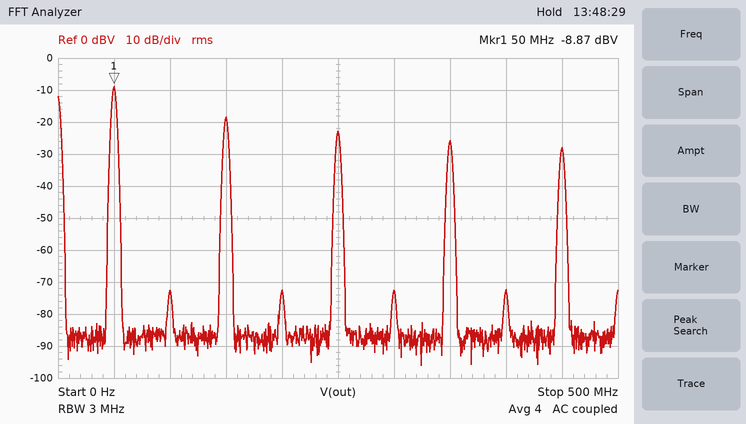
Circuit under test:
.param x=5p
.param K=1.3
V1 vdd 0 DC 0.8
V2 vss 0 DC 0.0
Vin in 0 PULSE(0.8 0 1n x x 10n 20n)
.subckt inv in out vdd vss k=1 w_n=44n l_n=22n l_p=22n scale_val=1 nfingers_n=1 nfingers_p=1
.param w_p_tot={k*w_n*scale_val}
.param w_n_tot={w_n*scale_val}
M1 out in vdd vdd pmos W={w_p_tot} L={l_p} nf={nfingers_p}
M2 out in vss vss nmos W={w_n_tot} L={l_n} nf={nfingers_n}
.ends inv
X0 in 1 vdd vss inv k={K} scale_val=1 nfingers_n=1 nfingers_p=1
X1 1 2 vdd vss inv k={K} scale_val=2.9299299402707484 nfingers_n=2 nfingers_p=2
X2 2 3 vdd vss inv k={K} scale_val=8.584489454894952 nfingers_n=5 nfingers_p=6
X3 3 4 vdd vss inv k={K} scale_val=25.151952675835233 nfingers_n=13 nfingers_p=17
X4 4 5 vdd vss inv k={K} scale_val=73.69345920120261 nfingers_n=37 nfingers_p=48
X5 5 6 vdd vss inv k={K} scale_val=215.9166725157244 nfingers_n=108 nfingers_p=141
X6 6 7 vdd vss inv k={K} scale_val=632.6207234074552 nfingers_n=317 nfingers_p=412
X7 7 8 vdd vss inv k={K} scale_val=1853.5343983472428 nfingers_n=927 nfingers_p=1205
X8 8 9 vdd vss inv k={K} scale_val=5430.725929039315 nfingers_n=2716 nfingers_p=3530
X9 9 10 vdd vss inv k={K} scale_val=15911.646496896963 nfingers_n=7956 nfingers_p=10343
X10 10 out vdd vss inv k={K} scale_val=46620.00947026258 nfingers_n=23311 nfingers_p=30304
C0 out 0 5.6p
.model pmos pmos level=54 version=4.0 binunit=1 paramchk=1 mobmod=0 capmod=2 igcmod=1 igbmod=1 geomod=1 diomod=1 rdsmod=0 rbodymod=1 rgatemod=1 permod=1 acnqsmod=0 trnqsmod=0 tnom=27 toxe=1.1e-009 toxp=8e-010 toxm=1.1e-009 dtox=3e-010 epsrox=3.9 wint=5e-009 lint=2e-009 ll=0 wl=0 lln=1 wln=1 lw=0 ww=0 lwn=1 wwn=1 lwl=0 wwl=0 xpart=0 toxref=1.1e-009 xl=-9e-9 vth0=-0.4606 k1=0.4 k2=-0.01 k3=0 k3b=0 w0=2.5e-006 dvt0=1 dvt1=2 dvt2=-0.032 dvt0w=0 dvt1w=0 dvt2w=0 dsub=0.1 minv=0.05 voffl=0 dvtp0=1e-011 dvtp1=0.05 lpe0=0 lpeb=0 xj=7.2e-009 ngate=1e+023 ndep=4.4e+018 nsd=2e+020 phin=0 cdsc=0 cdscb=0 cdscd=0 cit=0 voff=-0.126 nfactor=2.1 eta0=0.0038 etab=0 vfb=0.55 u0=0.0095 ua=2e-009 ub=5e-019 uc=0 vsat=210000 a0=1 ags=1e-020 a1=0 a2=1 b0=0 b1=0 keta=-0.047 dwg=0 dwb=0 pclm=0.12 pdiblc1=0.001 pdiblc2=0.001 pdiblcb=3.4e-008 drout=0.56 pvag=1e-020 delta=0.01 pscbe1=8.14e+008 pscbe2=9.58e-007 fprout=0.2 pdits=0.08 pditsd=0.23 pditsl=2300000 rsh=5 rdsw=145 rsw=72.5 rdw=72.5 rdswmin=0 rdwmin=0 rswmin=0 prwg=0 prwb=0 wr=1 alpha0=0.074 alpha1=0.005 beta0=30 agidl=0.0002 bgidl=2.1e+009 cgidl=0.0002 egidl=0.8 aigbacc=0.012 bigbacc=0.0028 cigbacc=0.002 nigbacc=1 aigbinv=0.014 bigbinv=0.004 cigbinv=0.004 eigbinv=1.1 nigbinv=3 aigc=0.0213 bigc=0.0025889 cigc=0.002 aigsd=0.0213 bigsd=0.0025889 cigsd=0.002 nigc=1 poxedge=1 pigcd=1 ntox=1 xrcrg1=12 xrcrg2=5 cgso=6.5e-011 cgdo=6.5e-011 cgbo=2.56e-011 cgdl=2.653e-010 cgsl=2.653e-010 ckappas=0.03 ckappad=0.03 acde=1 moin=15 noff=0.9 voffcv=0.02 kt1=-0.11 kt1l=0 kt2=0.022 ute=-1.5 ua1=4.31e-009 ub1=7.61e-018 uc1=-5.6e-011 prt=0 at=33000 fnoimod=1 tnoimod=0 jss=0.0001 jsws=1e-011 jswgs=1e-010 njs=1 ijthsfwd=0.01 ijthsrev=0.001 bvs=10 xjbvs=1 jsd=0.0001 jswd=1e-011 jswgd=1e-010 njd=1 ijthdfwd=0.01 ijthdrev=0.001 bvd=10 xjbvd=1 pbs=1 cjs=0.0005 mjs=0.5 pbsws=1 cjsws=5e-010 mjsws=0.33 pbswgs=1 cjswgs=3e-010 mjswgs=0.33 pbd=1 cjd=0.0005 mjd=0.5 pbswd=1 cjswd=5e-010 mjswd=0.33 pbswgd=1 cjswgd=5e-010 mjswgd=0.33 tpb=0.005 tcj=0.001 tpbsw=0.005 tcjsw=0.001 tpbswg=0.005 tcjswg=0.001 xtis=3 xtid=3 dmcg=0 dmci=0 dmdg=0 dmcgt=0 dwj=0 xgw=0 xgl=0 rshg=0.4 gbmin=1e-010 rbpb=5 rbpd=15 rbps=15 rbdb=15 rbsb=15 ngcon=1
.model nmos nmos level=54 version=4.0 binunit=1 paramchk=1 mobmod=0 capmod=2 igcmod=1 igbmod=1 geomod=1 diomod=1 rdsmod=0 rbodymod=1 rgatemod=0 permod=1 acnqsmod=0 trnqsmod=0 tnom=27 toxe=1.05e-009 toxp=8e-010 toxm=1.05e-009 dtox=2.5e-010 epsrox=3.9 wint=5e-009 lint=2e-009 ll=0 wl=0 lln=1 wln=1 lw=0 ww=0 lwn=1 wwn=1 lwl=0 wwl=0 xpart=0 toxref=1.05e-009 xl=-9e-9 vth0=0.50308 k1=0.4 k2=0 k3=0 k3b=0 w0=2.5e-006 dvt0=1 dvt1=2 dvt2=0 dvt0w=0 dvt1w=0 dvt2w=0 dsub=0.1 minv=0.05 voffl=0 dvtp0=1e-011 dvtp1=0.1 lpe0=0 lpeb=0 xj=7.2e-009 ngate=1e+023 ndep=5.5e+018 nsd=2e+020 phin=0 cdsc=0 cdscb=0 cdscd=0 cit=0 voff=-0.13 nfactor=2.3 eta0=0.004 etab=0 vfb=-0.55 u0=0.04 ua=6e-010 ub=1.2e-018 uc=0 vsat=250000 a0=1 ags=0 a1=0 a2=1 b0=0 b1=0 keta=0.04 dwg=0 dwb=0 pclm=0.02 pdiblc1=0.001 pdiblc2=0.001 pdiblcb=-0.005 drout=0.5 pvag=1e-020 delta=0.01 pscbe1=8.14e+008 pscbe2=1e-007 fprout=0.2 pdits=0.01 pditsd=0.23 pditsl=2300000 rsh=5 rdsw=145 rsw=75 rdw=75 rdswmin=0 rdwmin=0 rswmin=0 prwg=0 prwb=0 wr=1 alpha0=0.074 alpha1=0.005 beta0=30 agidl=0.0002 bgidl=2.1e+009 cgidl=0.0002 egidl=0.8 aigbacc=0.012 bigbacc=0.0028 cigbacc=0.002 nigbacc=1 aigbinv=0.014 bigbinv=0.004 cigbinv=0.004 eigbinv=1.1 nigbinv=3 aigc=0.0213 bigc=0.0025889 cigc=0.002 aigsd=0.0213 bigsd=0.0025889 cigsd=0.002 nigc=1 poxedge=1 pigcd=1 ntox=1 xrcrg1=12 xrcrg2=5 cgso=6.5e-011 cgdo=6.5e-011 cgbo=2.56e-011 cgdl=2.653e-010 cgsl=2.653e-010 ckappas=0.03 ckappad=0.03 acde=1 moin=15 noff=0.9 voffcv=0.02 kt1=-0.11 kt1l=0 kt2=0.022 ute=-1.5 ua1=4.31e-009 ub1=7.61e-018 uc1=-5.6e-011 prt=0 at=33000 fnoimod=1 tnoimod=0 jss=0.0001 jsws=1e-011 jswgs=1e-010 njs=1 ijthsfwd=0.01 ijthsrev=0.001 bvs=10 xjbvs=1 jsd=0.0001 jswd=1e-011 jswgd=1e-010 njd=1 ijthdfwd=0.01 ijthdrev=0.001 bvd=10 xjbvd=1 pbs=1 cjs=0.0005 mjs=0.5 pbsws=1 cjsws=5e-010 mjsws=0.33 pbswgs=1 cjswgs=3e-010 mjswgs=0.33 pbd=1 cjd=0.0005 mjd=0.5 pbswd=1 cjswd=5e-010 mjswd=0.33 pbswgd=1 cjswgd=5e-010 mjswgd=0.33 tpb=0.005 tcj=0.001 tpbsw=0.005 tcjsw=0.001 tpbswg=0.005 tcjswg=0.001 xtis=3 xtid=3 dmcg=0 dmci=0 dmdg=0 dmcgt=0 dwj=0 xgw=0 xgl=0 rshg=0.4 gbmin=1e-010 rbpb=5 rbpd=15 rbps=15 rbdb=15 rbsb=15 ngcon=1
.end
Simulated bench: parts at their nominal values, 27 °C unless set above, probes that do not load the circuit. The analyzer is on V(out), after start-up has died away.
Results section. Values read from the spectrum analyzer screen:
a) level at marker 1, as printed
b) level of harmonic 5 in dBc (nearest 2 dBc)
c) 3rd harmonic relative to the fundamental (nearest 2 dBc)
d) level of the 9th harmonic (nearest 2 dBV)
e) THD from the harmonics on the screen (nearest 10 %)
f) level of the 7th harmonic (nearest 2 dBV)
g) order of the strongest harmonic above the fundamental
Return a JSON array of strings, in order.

["-8.87 dBV", "-14 dBc", "-10 dBc", "-28 dBV", "40 %", "-26 dBV", "3"]
